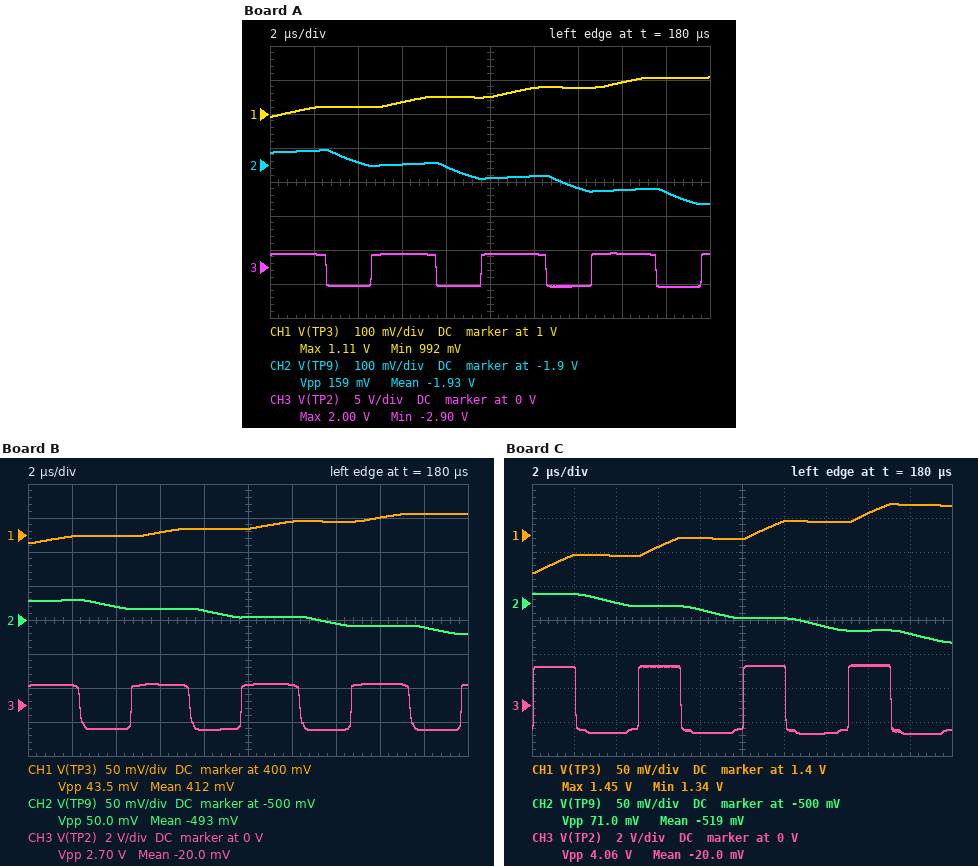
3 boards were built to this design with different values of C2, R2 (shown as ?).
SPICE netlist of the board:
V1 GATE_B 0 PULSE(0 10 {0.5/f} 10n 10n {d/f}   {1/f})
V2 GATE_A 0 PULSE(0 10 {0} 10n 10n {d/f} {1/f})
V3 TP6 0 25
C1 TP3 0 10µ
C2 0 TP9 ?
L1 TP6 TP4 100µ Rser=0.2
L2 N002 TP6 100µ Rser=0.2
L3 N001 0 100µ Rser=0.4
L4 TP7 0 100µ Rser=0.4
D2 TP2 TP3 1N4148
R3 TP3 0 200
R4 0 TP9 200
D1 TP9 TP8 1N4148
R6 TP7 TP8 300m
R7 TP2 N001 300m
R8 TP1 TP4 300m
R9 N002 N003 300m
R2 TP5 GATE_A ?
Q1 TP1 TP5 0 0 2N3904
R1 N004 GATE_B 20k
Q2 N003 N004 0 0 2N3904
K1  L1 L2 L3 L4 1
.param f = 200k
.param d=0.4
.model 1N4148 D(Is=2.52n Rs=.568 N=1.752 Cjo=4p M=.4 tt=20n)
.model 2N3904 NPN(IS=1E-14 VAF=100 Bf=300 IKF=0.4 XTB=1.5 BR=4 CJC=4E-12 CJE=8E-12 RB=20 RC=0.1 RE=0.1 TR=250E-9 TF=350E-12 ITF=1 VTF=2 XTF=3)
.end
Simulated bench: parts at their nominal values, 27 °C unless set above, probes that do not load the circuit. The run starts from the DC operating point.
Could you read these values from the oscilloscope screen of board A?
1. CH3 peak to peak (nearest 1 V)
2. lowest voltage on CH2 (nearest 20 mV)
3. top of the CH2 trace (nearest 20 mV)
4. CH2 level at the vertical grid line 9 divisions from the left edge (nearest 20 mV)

5 V
-2.02 V
-1.86 V
-1.98 V
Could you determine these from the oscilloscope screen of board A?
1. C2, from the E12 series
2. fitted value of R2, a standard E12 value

3.3 µF
27 kΩ
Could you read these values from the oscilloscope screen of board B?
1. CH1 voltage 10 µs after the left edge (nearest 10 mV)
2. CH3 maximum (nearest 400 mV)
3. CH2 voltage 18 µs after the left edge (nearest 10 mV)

410 mV
1.2 V
-510 mV
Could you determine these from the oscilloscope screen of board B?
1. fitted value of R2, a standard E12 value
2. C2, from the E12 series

68 kΩ
18 µF
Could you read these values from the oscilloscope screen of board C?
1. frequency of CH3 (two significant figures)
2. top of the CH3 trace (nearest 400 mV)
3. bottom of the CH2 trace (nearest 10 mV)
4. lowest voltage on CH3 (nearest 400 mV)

200 kHz
2.4 V
-560 mV
-1.6 V
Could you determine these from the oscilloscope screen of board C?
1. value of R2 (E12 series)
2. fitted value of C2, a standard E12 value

8.2 kΩ
33 µF
